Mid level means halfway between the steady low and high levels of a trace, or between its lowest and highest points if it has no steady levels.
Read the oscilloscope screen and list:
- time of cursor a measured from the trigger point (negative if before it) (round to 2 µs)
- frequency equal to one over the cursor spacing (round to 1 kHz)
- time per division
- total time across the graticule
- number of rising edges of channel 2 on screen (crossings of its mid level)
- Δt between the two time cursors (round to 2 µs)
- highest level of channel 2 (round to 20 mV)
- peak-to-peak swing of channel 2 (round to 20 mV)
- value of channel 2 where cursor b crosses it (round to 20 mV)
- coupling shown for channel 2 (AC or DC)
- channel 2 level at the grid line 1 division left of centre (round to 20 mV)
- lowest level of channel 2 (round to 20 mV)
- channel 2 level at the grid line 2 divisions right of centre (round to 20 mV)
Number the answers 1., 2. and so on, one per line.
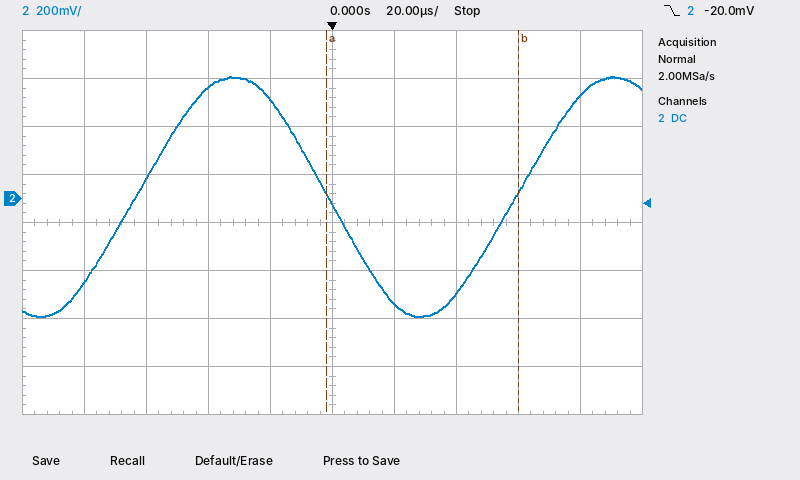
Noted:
1. -2 µs
2. 16 kHz
3. 20 µs
4. 200 µs
5. 2
6. 62 µs
7. 500 mV
8. 1.00 V
9. 20 mV
10. DC
11. 420 mV
12. -500 mV
13. -400 mV
